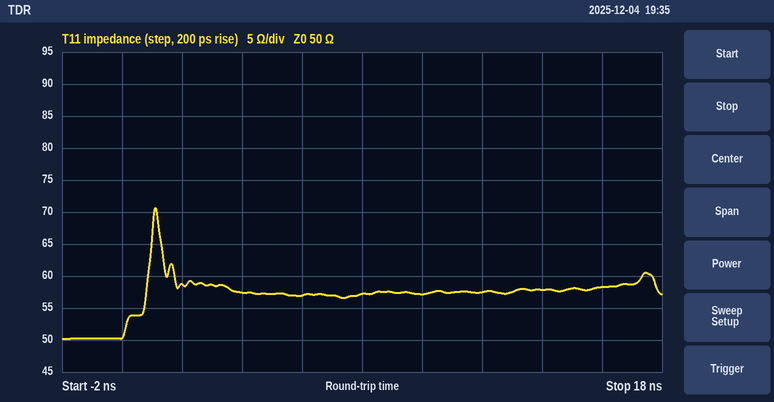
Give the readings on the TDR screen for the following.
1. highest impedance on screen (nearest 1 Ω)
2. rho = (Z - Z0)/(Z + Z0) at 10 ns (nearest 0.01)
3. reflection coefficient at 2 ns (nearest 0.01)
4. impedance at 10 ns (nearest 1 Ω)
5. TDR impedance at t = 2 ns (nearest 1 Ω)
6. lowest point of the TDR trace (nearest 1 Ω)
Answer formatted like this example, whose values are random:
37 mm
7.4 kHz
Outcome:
71 Ω
+0.07
+0.08
57 Ω
59 Ω
50 Ω
